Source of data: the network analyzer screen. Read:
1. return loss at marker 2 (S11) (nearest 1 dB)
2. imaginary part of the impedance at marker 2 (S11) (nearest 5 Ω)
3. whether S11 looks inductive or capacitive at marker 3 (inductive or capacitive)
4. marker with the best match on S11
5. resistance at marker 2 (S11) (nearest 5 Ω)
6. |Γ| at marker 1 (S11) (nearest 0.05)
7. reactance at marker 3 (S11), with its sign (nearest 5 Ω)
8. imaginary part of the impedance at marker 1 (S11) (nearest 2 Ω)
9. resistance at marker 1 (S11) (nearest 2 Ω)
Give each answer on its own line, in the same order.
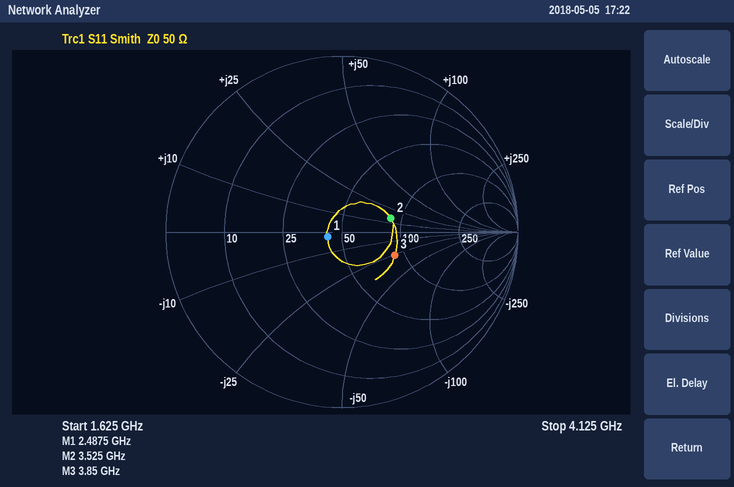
11 dB
+15 Ω
capacitive
marker 1
85 Ω
0.10
-25 Ω
-2 Ω
42 Ω
